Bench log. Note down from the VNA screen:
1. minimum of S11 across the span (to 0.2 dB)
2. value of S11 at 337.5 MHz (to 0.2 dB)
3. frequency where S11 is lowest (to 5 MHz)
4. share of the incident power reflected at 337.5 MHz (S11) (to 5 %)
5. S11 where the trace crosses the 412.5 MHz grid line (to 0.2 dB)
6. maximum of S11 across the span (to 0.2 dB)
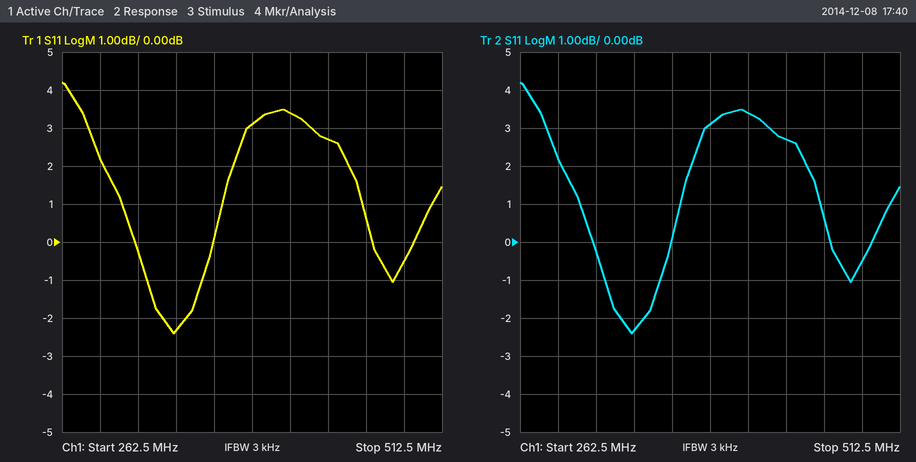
-2.4 dB
-2.4 dB
335 MHz
60 %
3.4 dB
4.2 dB
